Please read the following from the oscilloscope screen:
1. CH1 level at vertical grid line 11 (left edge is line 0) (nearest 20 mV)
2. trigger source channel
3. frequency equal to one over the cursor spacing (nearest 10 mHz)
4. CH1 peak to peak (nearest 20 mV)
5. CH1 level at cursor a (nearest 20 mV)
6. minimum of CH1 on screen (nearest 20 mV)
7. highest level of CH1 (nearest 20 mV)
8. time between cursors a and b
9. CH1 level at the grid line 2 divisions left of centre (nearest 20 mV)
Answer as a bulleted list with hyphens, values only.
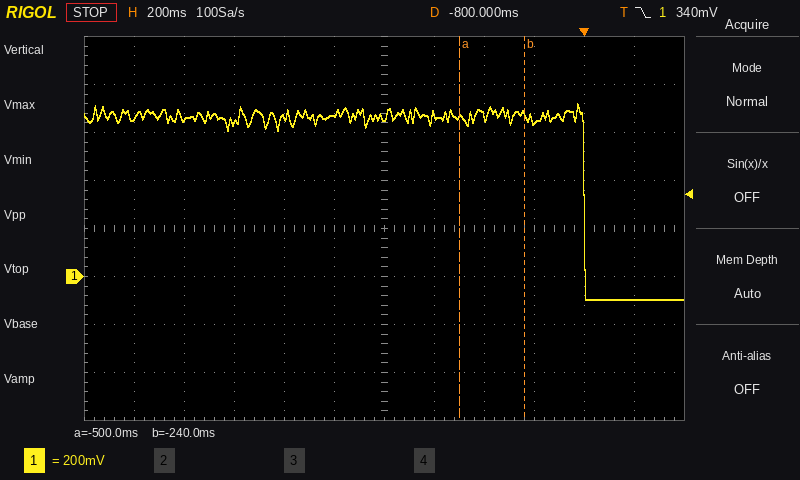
- -100 mV
- CH1
- 3.85 Hz
- 820 mV
- 660 mV
- -100 mV
- 720 mV
- 260 ms
- 660 mV
